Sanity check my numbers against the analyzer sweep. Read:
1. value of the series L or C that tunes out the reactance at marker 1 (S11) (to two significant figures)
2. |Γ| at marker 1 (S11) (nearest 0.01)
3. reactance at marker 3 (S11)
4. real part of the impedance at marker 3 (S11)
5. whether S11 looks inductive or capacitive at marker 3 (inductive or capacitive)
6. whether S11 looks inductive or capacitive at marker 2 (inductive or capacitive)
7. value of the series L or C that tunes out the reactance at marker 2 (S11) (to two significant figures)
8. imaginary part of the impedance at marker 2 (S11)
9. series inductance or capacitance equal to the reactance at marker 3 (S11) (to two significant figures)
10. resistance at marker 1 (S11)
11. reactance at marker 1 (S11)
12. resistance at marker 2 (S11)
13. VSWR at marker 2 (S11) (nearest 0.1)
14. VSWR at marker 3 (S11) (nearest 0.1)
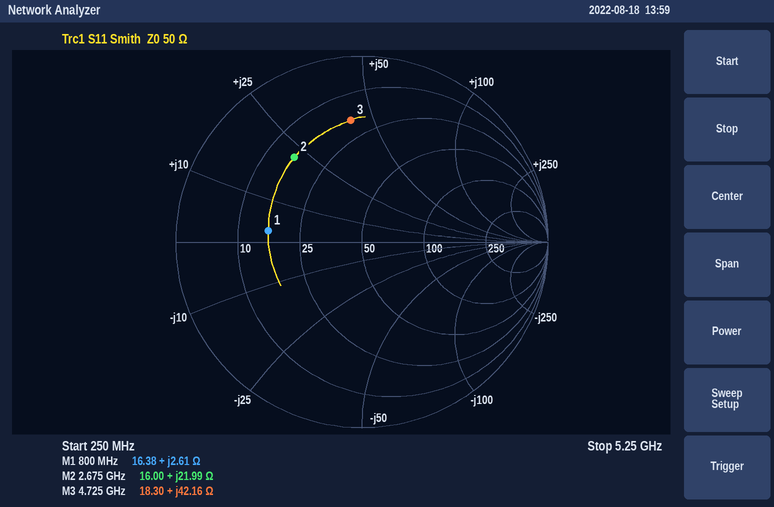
76 pF
0.51
+42.16 Ω
18.30 Ω
inductive
inductive
2.7 pF
+21.99 Ω
1.4 nH
16.38 Ω
+2.61 Ω
16.00 Ω
3.8
4.8
